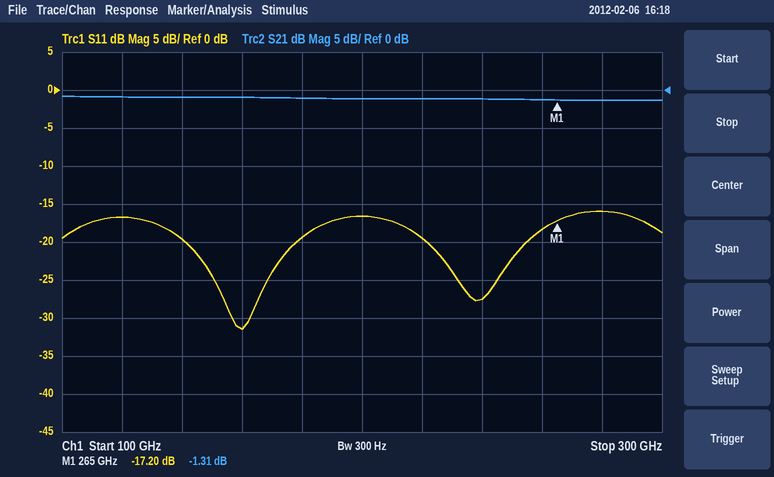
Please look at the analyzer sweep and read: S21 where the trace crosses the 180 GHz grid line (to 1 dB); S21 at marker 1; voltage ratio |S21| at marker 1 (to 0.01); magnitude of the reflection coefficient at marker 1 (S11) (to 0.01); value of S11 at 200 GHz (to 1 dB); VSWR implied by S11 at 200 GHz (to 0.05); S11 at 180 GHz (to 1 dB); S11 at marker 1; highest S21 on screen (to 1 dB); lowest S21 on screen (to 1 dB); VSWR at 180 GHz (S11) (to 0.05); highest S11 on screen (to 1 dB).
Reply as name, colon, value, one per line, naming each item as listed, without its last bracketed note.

S21 where the trace crosses the 180 GHz grid line: -1 dB
S21 at marker 1: -1.31 dB
voltage ratio |S21| at marker 1: 0.86
magnitude of the reflection coefficient at marker 1 (S11): 0.14
value of S11 at 200 GHz: -17 dB
VSWR implied by S11 at 200 GHz: 1.35
S11 at 180 GHz: -19 dB
S11 at marker 1: -17.20 dB
highest S21 on screen: -1 dB
lowest S21 on screen: -1 dB
VSWR at 180 GHz (S11): 1.25
highest S11 on screen: -16 dB
